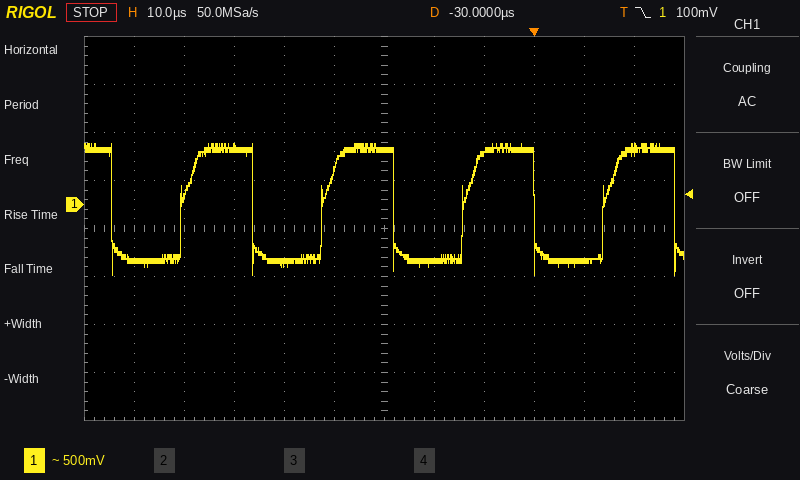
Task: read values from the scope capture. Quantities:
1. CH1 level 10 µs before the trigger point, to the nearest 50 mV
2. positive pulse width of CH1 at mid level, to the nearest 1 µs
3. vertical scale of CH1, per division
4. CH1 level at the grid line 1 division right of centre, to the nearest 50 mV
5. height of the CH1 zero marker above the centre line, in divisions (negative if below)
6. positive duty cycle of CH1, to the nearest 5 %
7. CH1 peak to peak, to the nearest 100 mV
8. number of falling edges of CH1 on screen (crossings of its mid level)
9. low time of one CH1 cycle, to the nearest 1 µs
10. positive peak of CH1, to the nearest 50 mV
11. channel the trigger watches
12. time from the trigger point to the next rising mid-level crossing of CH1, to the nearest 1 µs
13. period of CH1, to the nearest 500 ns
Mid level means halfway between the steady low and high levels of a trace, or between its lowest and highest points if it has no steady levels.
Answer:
550 mV
14 µs
500 mV
-600 mV
+0.5 div
50 %
1.40 V
5
14 µs
650 mV
CH1
14 µs
28.0 µs
